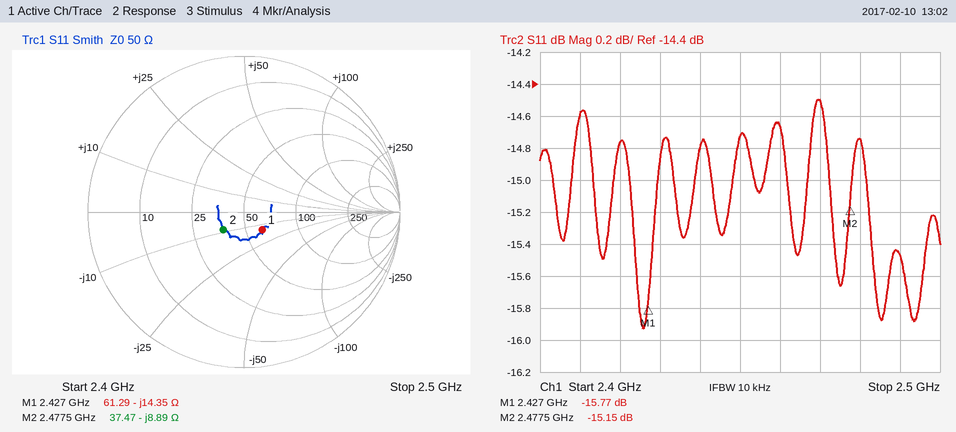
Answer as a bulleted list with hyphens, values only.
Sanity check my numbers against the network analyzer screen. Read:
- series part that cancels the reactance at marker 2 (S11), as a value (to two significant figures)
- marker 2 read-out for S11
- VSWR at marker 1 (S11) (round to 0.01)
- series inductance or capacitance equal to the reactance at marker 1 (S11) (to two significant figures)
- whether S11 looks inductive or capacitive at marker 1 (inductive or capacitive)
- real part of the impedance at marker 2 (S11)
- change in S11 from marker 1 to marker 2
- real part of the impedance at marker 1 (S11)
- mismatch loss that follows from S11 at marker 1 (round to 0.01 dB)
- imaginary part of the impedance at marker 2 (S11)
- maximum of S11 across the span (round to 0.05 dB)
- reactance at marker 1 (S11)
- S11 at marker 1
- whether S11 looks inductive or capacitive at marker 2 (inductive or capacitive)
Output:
- 570 pH
- -15.15 dB
- 1.39
- 4.6 pF
- capacitive
- 37.47 Ω
- 0.62 dB
- 61.29 Ω
- 0.12 dB
- -8.89 Ω
- -14.50 dB
- -14.35 Ω
- -15.77 dB
- capacitive
